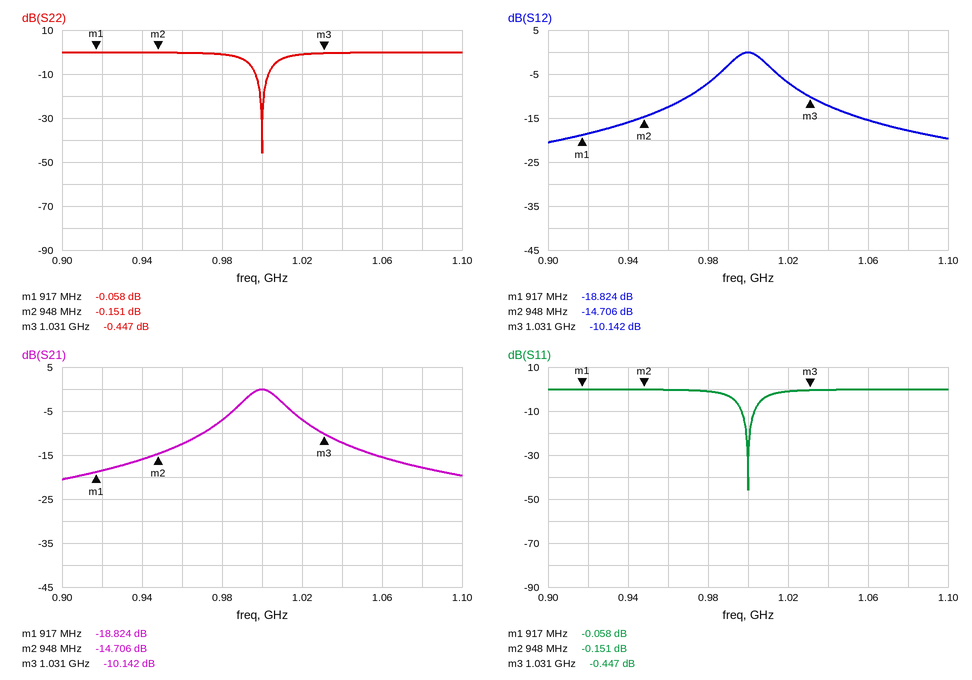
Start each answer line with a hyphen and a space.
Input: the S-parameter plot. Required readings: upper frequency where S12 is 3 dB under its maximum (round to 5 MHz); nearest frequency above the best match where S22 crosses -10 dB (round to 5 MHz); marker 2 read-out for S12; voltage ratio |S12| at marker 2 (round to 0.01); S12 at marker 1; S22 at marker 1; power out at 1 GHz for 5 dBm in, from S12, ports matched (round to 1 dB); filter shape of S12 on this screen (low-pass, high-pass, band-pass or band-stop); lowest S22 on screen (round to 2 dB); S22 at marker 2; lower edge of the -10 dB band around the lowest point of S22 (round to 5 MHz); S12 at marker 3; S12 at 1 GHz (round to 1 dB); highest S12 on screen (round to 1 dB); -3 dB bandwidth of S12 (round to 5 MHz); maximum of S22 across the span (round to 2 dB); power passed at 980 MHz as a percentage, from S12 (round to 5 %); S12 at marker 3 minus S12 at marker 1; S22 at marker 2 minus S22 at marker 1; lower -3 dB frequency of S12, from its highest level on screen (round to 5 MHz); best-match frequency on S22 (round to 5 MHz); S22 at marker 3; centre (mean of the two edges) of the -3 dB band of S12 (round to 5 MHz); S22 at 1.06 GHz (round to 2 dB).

- 1.010 GHz
- 1.005 GHz
- -14.706 dB
- 0.18
- -18.824 dB
- -0.058 dB
- 5 dBm
- band-pass
- -46 dB
- -0.151 dB
- 995 MHz
- -10.142 dB
- 0 dB
- 0 dB
- 20 MHz
- 0 dB
- 20 %
- 8.682 dB
- -0.093 dB
- 990 MHz
- 1.000 GHz
- -0.447 dB
- 1.000 GHz
- 0 dB
